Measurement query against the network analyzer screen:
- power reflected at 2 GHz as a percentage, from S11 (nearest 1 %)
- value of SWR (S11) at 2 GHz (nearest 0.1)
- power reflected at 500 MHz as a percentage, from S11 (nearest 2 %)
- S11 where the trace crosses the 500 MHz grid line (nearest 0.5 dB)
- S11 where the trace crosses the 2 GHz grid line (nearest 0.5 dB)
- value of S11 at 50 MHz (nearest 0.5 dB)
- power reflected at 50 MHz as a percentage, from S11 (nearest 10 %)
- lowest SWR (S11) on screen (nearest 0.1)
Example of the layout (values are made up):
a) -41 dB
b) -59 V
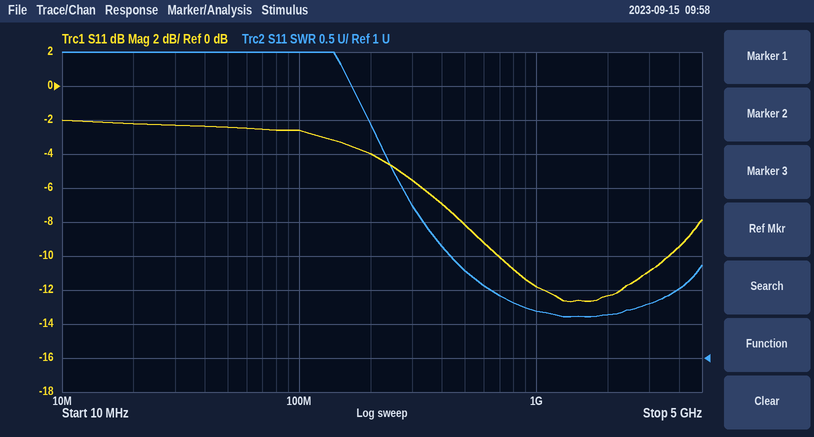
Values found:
a) 6 %
b) 1.6
c) 16 %
d) -8.0 dB
e) -12.5 dB
f) -2.5 dB
g) 60 %
h) 1.6
